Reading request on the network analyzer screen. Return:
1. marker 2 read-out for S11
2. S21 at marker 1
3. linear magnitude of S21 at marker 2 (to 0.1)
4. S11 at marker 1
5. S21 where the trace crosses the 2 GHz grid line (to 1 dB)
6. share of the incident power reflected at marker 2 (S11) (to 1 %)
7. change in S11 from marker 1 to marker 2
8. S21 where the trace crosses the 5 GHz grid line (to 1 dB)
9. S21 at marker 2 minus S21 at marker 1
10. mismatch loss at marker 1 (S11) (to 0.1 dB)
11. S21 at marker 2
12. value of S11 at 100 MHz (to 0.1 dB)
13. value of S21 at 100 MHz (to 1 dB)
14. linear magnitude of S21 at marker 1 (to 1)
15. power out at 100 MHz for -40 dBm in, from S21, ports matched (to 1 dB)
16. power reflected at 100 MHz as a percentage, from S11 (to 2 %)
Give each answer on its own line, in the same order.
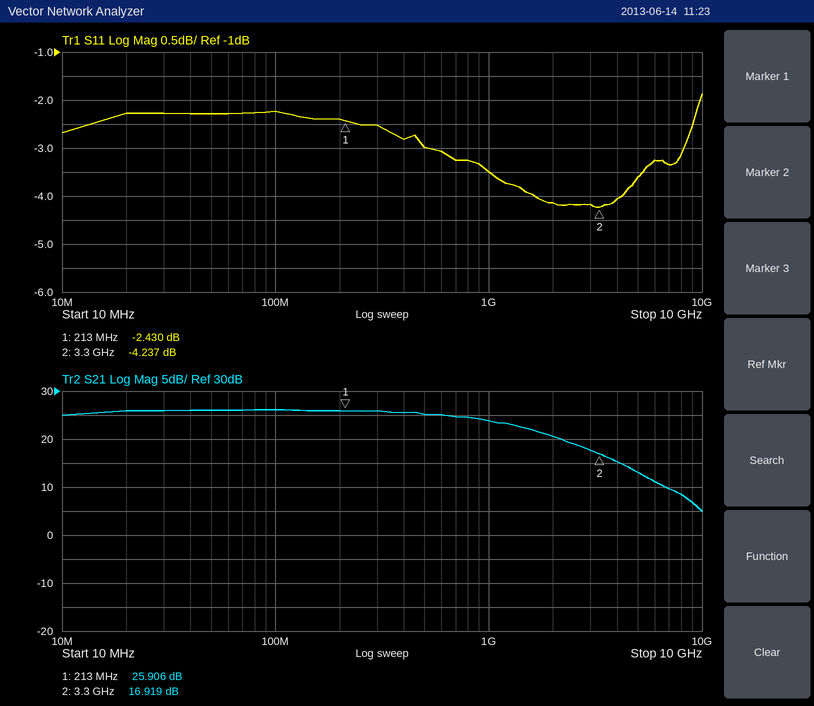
-4.237 dB
25.906 dB
7.0
-2.430 dB
21 dB
38 %
-1.807 dB
13 dB
-8.987 dB
3.7 dB
16.919 dB
-2.2 dB
26 dB
20
-14 dBm
60 %
